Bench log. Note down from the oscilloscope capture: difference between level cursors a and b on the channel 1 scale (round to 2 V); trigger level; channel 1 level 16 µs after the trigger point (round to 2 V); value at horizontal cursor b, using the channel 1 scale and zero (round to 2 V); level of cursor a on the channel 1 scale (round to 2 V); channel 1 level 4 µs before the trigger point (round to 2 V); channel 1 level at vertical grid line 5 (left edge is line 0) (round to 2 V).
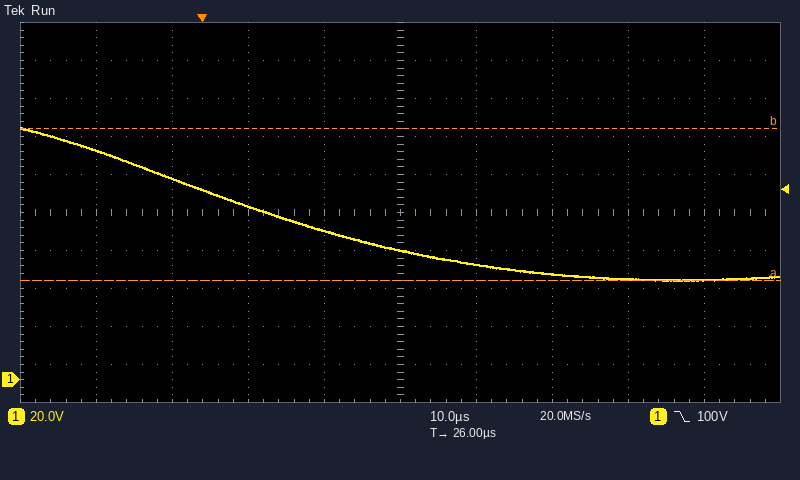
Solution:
80 V
100 V
78 V
132 V
52 V
106 V
68 V
